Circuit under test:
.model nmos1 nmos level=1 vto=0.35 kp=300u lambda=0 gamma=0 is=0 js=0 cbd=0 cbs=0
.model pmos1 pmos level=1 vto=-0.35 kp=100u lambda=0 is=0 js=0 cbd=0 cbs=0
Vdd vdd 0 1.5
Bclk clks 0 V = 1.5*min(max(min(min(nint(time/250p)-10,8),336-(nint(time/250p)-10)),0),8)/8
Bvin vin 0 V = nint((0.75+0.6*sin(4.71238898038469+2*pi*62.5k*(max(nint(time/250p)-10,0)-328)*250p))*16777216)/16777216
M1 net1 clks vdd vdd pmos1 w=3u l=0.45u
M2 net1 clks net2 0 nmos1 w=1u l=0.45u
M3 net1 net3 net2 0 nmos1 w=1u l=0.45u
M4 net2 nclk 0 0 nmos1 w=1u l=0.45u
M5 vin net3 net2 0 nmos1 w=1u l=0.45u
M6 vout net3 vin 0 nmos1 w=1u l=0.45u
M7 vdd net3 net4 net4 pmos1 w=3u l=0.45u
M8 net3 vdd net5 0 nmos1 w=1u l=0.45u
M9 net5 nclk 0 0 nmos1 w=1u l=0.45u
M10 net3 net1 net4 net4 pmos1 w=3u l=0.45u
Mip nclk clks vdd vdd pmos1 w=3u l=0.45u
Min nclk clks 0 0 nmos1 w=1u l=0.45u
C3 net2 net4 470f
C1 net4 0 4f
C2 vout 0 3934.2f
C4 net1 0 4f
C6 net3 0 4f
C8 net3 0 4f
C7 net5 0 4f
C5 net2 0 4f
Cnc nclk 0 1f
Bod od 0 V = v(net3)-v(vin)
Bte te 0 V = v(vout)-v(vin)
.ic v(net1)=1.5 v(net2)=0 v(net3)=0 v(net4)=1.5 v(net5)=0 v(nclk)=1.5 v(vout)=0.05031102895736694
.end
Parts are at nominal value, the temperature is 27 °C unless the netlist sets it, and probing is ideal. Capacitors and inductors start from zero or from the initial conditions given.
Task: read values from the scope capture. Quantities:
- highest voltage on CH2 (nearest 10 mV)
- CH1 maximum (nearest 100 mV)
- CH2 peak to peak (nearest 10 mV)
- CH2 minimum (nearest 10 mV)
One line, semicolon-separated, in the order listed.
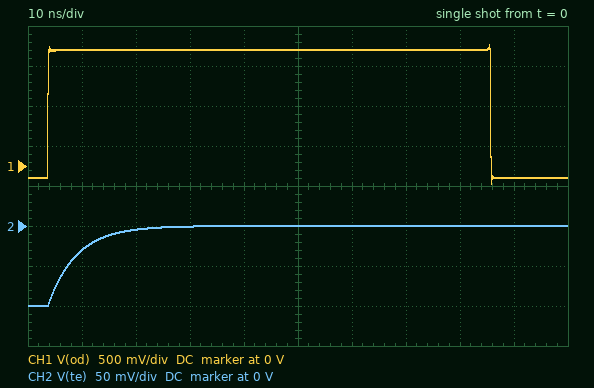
0 V; 1.5 V; 100 mV; -100 mV
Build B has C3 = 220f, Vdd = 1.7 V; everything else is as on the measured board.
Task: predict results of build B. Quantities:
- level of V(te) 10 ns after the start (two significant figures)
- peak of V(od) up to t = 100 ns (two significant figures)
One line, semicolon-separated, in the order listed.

-27 mV; 1.6 V
